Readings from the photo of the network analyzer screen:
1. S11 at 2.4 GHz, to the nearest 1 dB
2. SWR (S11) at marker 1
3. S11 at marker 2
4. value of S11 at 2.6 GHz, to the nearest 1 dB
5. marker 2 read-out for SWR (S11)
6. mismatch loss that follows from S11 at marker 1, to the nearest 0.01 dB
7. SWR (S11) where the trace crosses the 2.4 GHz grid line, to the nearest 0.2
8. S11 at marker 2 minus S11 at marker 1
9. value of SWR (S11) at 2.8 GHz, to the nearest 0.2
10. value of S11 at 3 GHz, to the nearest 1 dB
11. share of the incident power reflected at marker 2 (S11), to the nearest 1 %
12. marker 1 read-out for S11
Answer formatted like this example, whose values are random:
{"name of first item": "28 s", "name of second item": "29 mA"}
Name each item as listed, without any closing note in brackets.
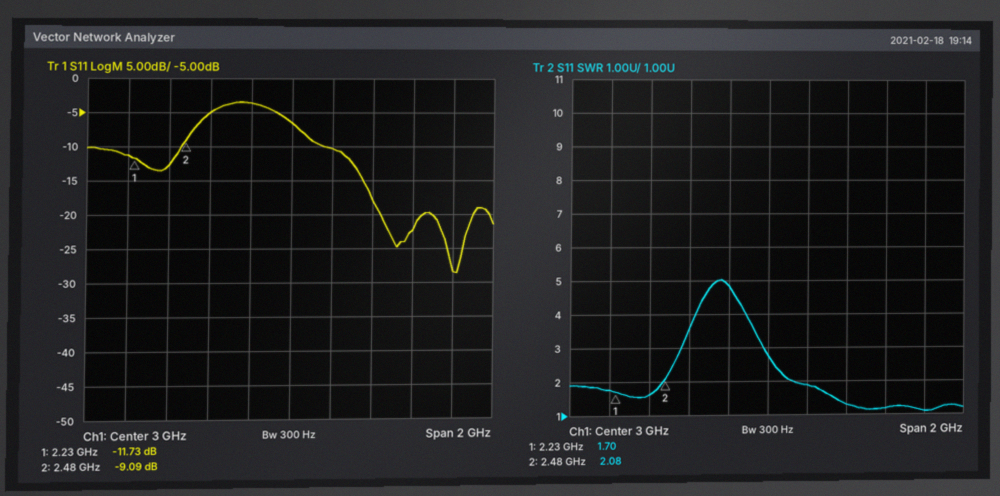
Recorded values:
{"S11 at 2.4 GHz, to the nearest 1 dB": "-13 dB", "SWR (S11) at marker 1": "1.70", "S11 at marker 2": "-9.09 dB", "value of S11 at 2.6 GHz, to the nearest 1 dB": "-5 dB", "marker 2 read-out for SWR": "2.08", "mismatch loss that follows from S11 at marker 1, to the nearest 0.01 dB": "0.30 dB", "SWR (S11) where the trace crosses the 2.4 GHz grid line, to the nearest 0.2": "1.6", "S11 at marker 2 minus S11 at marker 1": "2.64 dB", "value of SWR (S11) at 2.8 GHz, to the nearest 0.2": "4.8", "value of S11 at 3 GHz, to the nearest 1 dB": "-7 dB", "share of the incident power reflected at marker 2 (S11), to the nearest 1 %": "12 %", "marker 1 read-out for S11": "-11.73 dB"}
